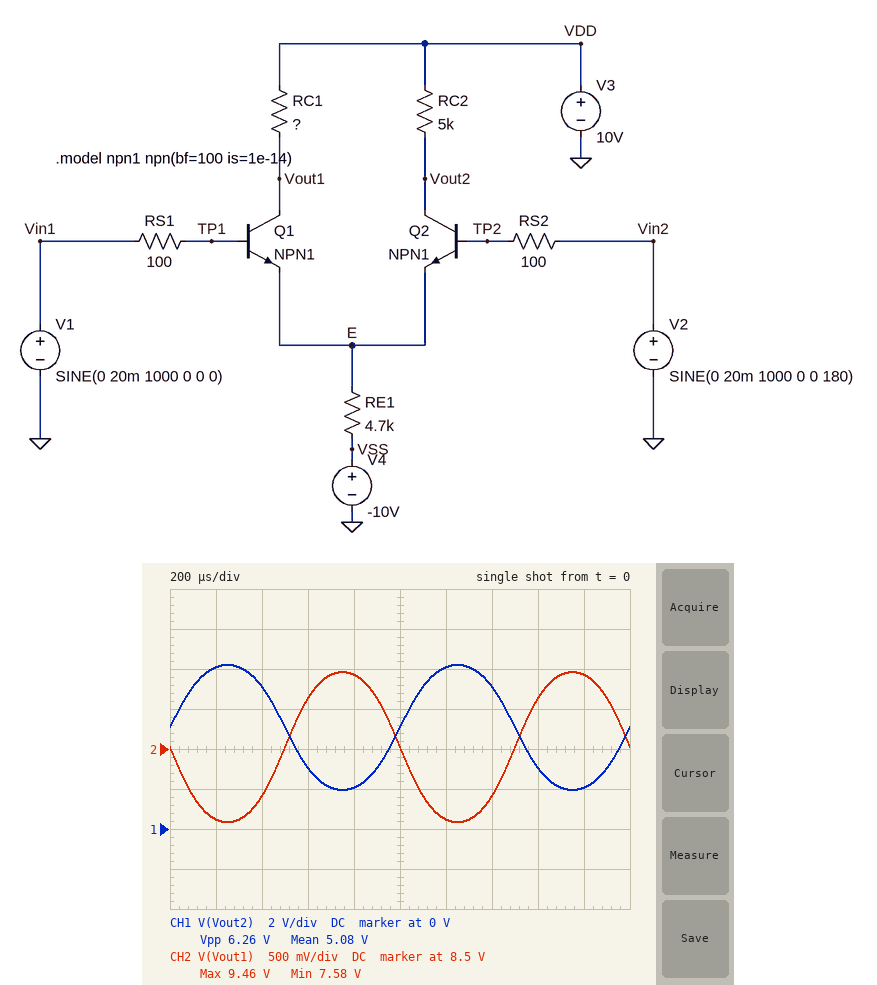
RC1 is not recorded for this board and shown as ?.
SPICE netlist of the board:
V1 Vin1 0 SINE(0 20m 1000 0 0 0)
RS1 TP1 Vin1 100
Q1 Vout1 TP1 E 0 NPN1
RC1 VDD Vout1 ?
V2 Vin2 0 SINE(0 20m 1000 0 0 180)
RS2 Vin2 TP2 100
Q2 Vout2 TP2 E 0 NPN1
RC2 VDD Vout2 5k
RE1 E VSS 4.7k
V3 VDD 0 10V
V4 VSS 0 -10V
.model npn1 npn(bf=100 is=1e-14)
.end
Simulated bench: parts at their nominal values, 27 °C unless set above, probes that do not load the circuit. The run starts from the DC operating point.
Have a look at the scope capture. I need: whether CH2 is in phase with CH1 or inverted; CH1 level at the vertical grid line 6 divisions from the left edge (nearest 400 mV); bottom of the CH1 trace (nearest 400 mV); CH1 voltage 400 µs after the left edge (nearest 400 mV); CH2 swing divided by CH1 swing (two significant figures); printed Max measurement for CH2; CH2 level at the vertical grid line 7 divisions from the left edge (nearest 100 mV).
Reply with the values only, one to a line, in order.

inverted
8.0 V
2.0 V
7.2 V
0.30
9.46 V
7.9 V
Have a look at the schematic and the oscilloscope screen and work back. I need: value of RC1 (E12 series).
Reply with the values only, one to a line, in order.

1.5 kΩ
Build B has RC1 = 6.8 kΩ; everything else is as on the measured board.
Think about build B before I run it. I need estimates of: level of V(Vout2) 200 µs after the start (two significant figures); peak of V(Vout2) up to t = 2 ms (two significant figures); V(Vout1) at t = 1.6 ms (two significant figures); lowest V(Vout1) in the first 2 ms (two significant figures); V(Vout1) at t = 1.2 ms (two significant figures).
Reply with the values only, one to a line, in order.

8.0 V
8.0 V
6.1 V
-540 mV
-530 mV
